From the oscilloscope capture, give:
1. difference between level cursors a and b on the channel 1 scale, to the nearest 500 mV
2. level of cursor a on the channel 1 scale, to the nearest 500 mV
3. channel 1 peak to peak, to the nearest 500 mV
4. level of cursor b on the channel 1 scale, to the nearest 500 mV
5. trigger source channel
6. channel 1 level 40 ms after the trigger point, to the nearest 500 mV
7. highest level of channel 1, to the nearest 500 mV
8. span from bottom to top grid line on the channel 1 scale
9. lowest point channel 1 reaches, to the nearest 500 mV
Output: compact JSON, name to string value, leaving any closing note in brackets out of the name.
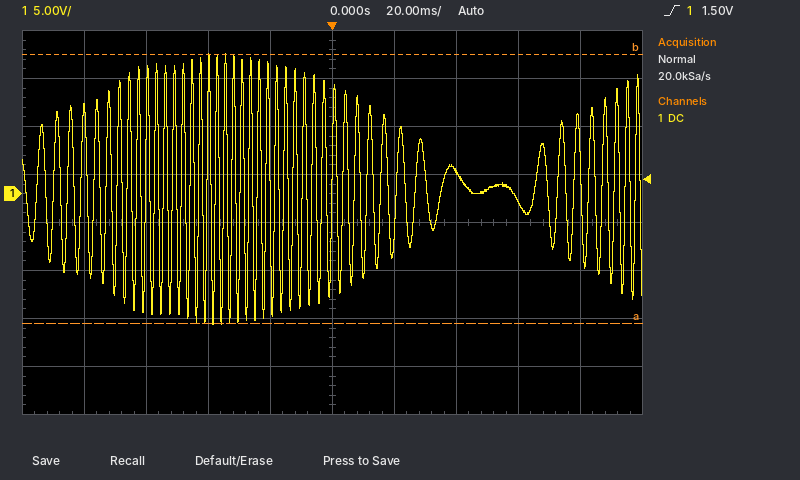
{"difference between level cursors a and b on the channel 1 scale, to the nearest 500 mV": "28.0 V", "level of cursor a on the channel 1 scale, to the nearest 500 mV": "-13.5 V", "channel 1 peak to peak, to the nearest 500 mV": "28.0 V", "level of cursor b on the channel 1 scale, to the nearest 500 mV": "14.5 V", "trigger source channel": "channel 1", "channel 1 level 40 ms after the trigger point, to the nearest 500 mV": "2.5 V", "highest level of channel 1, to the nearest 500 mV": "14.5 V", "span from bottom to top grid line on the channel 1 scale": "40 V", "lowest point channel 1 reaches, to the nearest 500 mV": "-13.5 V"}
